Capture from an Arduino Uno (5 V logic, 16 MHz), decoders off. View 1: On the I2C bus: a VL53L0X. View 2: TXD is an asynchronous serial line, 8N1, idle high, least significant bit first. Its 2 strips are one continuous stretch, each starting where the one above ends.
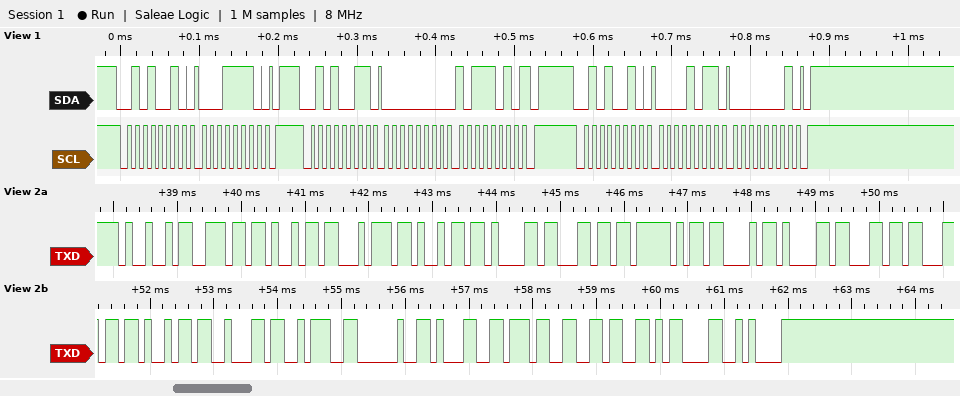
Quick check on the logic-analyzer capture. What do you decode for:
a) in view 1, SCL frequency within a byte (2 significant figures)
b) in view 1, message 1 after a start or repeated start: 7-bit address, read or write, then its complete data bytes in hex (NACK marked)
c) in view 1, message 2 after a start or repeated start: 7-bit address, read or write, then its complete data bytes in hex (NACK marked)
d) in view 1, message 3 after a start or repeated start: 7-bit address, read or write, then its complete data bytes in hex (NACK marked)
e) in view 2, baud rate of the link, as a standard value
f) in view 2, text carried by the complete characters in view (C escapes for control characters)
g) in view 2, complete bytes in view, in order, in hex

100 kHz
0x29 write: 1E
0x29 read: 00 BA NACK
0x29 write: 0B 01
9600 baud
"Initial_Callib: 176\r\n"
49 6E 69 74 69 61 6C 5F 43 61 6C 6C 69 62 3A 20 31 37 36 0D 0A
